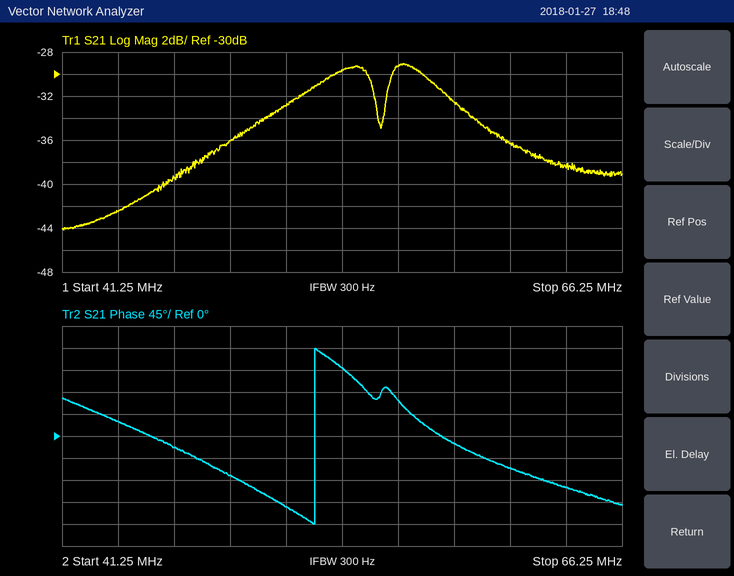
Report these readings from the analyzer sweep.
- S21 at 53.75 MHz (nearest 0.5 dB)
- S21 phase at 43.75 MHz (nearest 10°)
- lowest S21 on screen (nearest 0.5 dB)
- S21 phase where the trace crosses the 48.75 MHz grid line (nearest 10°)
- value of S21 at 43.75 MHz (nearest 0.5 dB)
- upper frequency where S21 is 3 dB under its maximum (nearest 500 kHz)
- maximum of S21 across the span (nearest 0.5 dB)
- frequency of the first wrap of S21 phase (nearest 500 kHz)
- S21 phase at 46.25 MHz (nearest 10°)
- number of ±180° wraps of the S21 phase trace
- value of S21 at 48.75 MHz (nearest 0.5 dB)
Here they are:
-29.5 dB
30°
-44.0 dB
-80°
-42.5 dB
58.5 MHz
-29.0 dB
52.5 MHz
-20°
1
-36.0 dB
